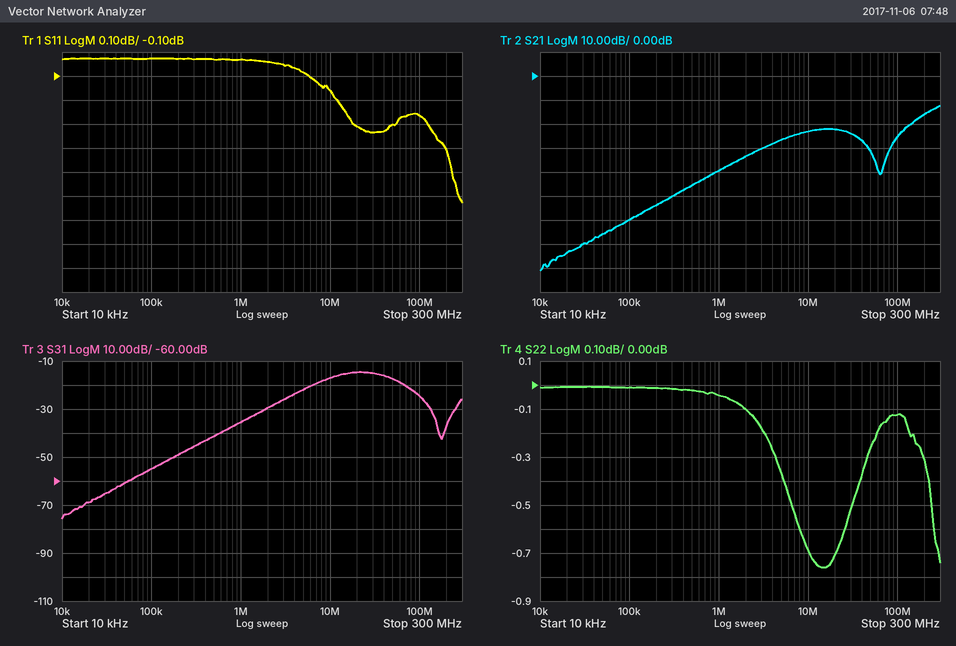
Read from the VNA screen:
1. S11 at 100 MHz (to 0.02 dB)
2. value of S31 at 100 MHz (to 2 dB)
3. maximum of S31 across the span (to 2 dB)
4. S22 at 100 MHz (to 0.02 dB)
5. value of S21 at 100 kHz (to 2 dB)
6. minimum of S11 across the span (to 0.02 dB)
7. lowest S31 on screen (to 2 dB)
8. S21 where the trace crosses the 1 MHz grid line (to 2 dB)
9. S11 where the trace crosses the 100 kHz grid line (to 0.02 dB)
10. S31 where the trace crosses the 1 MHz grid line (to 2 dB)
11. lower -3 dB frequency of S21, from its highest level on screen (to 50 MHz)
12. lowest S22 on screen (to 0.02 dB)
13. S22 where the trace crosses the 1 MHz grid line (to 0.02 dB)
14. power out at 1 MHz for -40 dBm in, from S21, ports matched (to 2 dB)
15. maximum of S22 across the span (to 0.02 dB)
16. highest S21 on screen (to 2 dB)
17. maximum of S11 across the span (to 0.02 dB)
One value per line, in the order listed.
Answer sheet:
-0.26 dB
-24 dB
-14 dB
-0.12 dB
-60 dB
-0.62 dB
-76 dB
-40 dB
-0.02 dB
-36 dB
200 MHz
-0.76 dB
-0.04 dB
-80 dBm
0.00 dB
-12 dB
-0.02 dB
